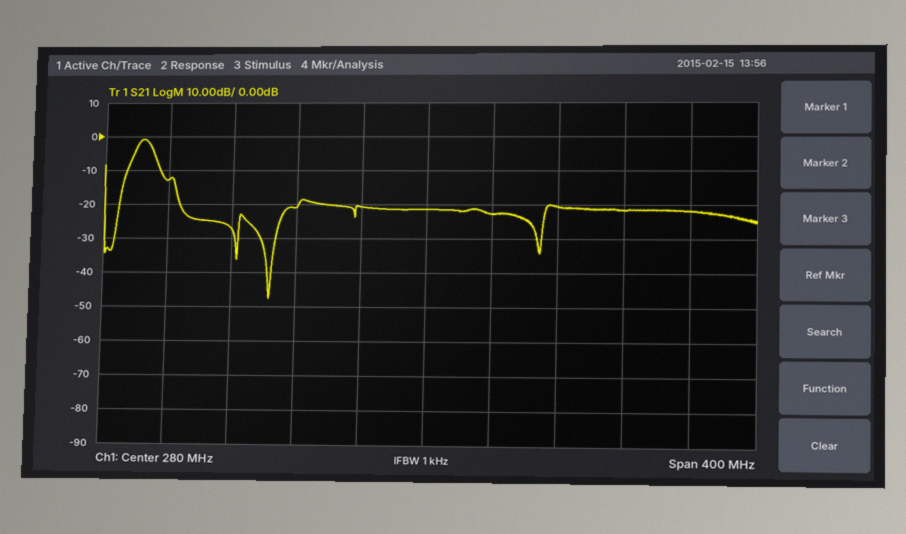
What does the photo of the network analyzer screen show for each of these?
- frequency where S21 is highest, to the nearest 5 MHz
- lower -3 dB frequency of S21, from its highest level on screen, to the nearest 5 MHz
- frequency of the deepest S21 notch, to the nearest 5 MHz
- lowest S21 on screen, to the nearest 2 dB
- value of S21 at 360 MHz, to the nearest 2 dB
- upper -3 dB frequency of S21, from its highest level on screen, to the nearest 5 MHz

105 MHz
100 MHz
185 MHz
-48 dB
-20 dB
110 MHz
